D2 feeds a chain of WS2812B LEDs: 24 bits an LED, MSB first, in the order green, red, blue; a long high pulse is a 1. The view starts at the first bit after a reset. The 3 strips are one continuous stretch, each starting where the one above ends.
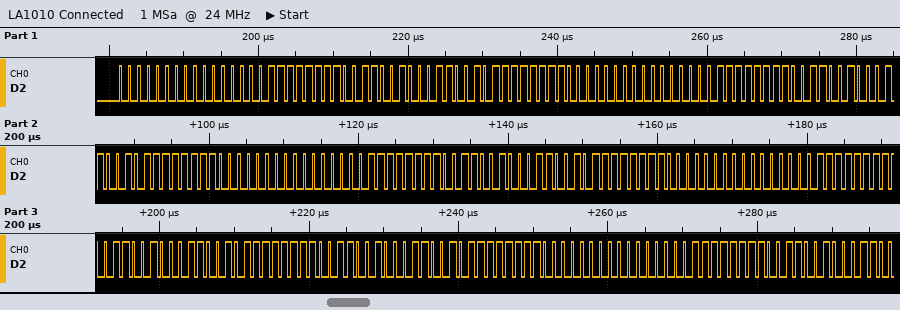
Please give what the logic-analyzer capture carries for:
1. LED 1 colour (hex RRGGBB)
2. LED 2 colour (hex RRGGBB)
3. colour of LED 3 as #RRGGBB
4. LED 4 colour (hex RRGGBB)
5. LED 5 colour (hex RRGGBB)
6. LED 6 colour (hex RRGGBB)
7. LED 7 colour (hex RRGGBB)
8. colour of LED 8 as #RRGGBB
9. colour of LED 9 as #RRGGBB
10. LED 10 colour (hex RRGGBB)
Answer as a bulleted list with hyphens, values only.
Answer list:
- #0000FF
- #3232FF
- #0000FF
- #3232FF
- #0000FF
- #3232FF
- #0000FF
- #3232FF
- #3232FF
- #0000FF
